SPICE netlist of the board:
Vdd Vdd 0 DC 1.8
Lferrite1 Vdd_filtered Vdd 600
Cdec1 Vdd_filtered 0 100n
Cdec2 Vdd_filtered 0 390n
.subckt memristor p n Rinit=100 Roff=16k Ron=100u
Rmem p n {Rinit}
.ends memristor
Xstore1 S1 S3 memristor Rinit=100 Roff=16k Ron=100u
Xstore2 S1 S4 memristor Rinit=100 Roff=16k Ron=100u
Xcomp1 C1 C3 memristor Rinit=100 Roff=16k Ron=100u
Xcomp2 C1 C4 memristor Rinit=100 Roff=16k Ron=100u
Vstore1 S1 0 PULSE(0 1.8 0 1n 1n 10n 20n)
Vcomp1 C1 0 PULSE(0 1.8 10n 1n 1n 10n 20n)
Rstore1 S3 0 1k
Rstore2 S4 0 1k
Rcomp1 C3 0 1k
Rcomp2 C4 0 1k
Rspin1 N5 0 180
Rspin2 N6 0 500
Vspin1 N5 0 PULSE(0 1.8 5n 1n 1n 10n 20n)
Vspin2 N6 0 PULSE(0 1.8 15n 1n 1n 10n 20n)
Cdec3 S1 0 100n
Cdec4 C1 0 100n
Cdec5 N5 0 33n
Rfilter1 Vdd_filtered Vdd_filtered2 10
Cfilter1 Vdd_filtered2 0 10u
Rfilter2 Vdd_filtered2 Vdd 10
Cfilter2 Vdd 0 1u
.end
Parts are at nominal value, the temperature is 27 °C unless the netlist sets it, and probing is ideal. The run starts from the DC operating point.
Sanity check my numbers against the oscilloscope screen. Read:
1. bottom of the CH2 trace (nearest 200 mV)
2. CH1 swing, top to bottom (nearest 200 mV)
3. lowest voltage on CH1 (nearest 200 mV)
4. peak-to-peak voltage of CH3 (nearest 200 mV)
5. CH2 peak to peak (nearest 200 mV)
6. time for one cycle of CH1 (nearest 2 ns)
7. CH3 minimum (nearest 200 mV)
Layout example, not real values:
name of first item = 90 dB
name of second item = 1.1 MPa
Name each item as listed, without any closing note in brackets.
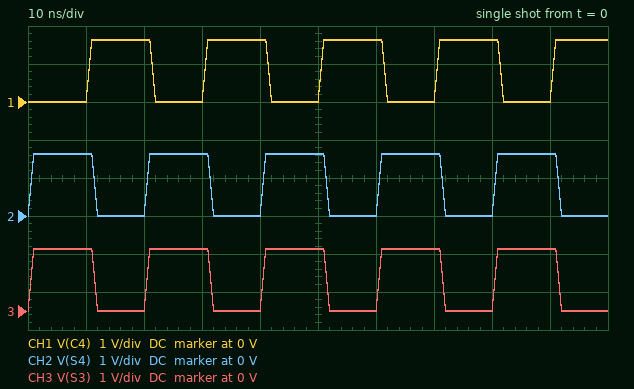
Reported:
bottom of the CH2 trace = 0 V
CH1 swing, top to bottom = 1.6 V
lowest voltage on CH1 = 0 V
peak-to-peak voltage of CH3 = 1.6 V
CH2 peak to peak = 1.6 V
time for one cycle of CH1 = 20 ns
CH3 minimum = 0 V
